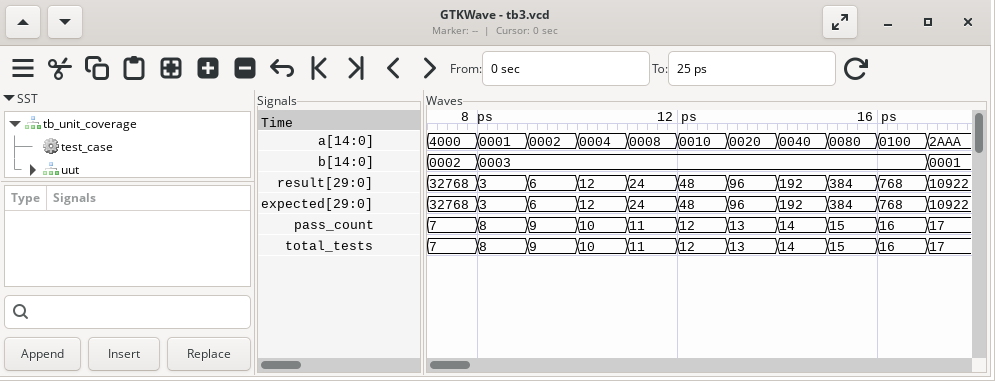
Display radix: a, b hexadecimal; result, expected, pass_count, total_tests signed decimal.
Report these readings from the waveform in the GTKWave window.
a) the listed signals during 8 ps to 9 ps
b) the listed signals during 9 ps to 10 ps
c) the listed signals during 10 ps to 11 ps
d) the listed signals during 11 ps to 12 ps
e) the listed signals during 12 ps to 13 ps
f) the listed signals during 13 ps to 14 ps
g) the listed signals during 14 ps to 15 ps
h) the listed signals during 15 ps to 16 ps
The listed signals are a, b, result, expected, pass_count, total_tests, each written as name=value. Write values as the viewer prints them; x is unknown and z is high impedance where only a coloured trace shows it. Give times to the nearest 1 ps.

a=0001, b=0003, result=3, expected=3, pass_count=8, total_tests=8
a=0002, b=0003, result=6, expected=6, pass_count=9, total_tests=9
a=0004, b=0003, result=12, expected=12, pass_count=10, total_tests=10
a=0008, b=0003, result=24, expected=24, pass_count=11, total_tests=11
a=0010, b=0003, result=48, expected=48, pass_count=12, total_tests=12
a=0020, b=0003, result=96, expected=96, pass_count=13, total_tests=13
a=0040, b=0003, result=192, expected=192, pass_count=14, total_tests=14
a=0080, b=0003, result=384, expected=384, pass_count=15, total_tests=15
